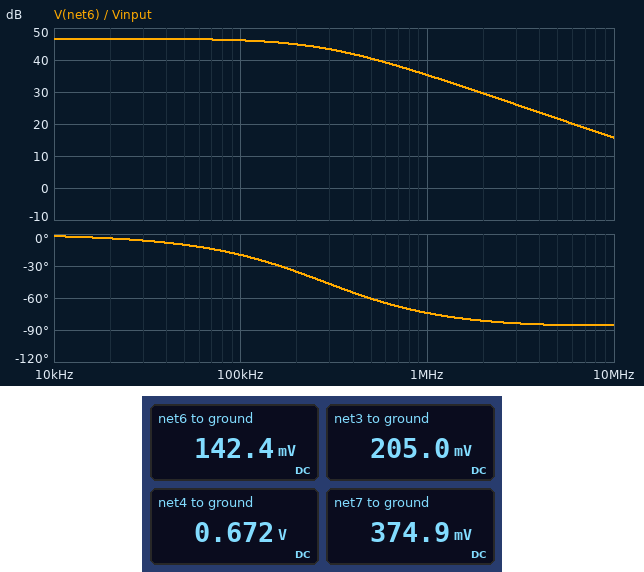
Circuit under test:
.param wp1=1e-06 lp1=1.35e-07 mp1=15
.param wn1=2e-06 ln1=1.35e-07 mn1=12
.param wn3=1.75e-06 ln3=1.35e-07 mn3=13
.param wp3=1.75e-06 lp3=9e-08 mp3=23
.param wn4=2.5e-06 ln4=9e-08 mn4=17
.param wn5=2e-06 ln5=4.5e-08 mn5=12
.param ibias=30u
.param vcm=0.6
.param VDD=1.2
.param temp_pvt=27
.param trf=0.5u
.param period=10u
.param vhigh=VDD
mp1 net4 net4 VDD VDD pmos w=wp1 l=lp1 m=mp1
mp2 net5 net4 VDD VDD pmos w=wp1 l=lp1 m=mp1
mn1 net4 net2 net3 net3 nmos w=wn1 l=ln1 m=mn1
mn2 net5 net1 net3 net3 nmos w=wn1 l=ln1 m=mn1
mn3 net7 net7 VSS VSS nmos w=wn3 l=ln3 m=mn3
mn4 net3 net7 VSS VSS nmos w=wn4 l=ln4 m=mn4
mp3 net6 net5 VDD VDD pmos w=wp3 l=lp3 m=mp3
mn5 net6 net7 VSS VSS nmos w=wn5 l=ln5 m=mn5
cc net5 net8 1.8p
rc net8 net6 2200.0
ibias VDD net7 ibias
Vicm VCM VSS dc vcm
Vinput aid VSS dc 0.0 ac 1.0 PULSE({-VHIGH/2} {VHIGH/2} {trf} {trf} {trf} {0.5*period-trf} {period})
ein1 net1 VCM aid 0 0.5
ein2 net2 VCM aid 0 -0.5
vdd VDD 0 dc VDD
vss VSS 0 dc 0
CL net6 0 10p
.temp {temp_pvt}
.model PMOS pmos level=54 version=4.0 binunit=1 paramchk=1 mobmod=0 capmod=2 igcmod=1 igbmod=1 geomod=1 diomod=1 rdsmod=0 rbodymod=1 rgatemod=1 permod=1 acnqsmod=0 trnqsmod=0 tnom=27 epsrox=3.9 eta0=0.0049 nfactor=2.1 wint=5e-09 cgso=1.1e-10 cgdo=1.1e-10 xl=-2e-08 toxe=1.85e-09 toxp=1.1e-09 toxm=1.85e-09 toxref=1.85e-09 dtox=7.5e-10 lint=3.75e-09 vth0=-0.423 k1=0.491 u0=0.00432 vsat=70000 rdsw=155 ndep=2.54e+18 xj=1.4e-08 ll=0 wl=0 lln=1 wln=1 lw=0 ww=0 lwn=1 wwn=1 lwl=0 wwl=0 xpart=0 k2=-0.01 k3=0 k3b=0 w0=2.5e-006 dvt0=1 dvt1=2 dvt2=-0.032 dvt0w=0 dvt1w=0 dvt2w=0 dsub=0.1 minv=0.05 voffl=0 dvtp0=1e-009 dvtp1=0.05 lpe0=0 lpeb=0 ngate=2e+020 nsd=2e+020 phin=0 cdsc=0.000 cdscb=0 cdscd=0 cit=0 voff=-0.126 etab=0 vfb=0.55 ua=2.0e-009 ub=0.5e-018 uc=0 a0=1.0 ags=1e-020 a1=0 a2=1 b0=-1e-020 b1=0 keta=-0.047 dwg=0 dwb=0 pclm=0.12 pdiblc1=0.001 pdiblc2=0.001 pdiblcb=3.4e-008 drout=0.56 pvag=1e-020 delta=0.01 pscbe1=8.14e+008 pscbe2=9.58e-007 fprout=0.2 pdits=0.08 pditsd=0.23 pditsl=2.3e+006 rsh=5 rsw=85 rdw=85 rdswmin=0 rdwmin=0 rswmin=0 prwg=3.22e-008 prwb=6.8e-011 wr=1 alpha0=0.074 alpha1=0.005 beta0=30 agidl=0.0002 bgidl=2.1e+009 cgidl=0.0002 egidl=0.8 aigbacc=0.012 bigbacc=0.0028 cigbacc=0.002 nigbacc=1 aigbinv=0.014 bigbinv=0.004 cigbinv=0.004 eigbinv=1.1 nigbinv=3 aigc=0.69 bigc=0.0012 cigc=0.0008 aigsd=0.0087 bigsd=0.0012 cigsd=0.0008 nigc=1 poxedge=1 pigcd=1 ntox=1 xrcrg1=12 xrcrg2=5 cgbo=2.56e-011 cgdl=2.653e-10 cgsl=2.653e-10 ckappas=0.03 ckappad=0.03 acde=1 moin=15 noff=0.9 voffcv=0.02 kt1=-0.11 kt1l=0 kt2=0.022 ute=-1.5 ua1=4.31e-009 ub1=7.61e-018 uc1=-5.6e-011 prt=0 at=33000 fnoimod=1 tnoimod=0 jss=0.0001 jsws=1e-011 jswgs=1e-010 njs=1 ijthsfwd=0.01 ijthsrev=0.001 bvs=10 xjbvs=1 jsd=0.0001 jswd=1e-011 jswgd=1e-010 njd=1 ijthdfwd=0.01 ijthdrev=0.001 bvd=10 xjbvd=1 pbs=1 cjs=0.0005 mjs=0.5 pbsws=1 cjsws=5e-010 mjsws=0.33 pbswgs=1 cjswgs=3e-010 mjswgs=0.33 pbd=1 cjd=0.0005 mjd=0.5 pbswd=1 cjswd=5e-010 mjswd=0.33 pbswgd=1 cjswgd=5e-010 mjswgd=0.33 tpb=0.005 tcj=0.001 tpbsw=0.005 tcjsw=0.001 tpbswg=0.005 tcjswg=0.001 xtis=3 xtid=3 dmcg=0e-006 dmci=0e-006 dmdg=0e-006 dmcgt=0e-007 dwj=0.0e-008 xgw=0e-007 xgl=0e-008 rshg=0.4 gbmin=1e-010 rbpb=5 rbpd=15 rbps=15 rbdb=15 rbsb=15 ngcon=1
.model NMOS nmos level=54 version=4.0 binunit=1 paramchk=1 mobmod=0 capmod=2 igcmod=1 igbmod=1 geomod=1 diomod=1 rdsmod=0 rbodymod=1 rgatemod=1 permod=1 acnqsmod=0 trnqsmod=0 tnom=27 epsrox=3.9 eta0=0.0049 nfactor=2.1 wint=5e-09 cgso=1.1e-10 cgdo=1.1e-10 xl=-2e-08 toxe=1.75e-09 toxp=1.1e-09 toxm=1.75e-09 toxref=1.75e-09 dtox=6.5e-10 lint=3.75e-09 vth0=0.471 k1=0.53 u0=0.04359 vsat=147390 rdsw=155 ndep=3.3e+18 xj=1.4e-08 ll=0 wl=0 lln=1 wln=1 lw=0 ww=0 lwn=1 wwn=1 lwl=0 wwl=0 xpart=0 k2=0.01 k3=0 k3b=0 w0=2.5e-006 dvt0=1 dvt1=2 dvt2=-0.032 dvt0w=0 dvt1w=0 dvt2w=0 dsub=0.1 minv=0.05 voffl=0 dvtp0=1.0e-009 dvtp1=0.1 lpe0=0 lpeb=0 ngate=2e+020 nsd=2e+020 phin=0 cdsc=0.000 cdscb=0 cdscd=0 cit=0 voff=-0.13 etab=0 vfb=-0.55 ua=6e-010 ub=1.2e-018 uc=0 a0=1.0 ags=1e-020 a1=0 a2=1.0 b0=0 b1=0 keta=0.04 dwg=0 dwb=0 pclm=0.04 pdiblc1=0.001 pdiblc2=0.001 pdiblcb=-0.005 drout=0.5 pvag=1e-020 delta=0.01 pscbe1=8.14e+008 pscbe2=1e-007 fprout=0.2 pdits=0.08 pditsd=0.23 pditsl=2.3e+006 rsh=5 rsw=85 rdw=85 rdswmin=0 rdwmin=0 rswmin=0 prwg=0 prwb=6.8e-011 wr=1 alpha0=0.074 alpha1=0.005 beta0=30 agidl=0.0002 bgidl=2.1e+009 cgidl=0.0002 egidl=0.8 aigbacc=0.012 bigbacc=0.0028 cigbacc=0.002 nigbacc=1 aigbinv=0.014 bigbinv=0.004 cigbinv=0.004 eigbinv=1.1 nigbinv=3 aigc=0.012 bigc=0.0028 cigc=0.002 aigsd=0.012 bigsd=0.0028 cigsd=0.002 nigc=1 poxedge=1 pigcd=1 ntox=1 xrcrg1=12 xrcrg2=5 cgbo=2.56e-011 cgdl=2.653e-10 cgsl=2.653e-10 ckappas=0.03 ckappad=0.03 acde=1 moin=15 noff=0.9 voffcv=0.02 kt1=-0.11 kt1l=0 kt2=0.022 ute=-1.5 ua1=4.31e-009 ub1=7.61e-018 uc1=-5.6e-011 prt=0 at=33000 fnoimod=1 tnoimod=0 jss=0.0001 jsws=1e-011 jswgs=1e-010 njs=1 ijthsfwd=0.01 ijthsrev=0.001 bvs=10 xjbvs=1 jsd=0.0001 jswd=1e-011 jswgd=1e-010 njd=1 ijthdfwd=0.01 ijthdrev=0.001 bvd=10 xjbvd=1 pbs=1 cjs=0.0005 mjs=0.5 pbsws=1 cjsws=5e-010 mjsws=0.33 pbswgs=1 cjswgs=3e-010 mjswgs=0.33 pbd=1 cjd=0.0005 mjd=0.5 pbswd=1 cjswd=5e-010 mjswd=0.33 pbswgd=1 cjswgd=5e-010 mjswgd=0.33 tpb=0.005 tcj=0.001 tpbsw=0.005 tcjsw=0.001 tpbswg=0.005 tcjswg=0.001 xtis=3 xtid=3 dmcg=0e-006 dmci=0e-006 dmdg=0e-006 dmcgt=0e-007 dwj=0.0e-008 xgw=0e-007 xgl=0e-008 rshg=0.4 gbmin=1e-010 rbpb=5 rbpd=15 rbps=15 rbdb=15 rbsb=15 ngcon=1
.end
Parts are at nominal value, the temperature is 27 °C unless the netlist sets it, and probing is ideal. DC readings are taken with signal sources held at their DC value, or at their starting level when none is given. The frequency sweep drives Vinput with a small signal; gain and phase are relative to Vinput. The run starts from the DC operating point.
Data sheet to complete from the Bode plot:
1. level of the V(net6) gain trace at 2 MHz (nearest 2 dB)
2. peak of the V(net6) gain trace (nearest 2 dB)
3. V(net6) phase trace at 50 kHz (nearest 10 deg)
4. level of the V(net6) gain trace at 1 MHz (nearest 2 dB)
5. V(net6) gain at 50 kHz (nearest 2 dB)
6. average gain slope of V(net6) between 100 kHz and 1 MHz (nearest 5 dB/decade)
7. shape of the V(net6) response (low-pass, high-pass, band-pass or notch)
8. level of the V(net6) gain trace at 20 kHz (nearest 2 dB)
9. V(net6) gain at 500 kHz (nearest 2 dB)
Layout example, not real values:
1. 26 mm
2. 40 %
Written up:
1. 30 dB
2. 46 dB
3. -10 deg
4. 36 dB
5. 46 dB
6. -10 dB/decade
7. low-pass
8. 46 dB
9. 40 dB
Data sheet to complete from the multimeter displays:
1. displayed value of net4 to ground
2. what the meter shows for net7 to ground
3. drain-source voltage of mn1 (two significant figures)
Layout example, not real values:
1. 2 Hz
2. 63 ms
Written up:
1. 0.672 V
2. 374.9 mV
3. 470 mV
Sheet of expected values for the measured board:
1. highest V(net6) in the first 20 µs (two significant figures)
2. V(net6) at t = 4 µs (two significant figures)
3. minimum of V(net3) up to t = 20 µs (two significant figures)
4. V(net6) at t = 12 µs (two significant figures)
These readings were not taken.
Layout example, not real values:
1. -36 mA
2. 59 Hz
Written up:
1. 1.0 V
2. 1.0 V
3. 4.9 mV
4. 1.0 V
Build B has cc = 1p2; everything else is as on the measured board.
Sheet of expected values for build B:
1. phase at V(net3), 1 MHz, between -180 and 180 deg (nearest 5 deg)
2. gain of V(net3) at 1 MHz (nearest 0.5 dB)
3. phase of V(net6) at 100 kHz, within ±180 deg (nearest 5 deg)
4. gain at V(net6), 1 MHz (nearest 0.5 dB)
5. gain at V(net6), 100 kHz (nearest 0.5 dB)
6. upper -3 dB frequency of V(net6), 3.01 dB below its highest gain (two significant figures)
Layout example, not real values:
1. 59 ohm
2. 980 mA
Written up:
1. 120 deg
2. -20.0 dB
3. -15 deg
4. 38.5 dB
5. 46.5 dB
6. 410 kHz
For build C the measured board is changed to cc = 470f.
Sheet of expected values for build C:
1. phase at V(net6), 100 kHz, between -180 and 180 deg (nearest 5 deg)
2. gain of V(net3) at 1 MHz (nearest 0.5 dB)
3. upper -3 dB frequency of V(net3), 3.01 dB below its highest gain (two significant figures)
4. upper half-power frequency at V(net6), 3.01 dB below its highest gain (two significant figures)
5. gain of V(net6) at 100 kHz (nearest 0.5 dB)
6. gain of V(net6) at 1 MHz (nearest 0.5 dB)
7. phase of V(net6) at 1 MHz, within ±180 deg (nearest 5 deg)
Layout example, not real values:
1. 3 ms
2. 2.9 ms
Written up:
1. -5 deg
2. -14.5 dB
3. 1.0 MHz
4. 990 kHz
5. 46.5 dB
6. 43.5 dB
7. -45 deg
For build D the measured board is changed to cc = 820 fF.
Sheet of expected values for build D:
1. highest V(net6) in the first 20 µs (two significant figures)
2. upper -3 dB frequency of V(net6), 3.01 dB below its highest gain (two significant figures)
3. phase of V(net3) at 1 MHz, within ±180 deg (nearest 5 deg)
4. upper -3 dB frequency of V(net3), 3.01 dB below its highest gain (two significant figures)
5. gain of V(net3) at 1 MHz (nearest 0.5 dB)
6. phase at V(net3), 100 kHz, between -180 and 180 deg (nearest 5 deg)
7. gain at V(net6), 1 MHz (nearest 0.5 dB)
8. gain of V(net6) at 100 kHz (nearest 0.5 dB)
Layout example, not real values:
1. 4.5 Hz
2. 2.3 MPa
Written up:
1. 1.0 V
2. 590 kHz
3. 130 deg
4. 600 kHz
5. -17.5 dB
6. 170 deg
7. 41.0 dB
8. 46.5 dB
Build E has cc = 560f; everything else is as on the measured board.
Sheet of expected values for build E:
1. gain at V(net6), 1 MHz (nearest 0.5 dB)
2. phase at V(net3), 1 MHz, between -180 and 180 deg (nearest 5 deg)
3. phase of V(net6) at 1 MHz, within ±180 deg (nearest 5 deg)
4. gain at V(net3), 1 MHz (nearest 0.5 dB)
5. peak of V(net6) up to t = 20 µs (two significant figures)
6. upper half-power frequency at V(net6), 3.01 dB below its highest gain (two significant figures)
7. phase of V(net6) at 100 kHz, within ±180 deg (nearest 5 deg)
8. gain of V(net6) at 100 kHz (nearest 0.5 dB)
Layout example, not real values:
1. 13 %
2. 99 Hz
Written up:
1. 43.0 dB
2. 140 deg
3. -50 deg
4. -15.5 dB
5. 1.0 V
6. 840 kHz
7. -5 deg
8. 46.5 dB
